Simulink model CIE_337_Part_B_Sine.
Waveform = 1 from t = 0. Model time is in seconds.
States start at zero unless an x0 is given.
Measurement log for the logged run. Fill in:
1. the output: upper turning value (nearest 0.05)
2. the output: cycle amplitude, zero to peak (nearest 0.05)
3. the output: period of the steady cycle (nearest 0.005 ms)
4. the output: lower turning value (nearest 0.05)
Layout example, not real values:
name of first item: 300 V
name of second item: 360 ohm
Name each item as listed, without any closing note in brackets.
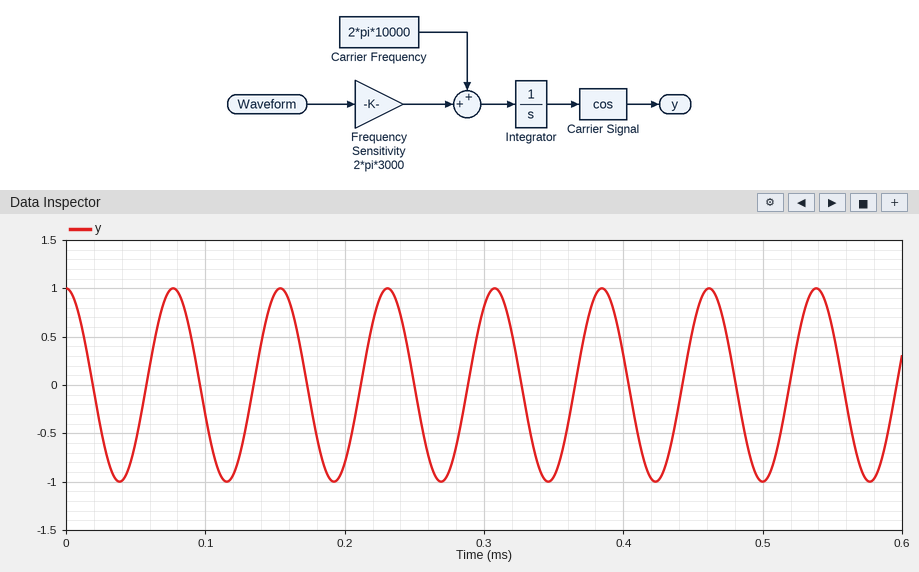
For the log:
the output: upper turning value: 1.00
the output: cycle amplitude, zero to peak: 1.00
the output: period of the steady cycle: 0.075 ms
the output: lower turning value: -1.00
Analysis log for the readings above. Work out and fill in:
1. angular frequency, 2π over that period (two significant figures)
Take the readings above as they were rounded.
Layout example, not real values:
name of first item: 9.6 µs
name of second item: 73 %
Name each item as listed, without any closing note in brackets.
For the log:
angular frequency, 2π over that period: 84 rad/ms
